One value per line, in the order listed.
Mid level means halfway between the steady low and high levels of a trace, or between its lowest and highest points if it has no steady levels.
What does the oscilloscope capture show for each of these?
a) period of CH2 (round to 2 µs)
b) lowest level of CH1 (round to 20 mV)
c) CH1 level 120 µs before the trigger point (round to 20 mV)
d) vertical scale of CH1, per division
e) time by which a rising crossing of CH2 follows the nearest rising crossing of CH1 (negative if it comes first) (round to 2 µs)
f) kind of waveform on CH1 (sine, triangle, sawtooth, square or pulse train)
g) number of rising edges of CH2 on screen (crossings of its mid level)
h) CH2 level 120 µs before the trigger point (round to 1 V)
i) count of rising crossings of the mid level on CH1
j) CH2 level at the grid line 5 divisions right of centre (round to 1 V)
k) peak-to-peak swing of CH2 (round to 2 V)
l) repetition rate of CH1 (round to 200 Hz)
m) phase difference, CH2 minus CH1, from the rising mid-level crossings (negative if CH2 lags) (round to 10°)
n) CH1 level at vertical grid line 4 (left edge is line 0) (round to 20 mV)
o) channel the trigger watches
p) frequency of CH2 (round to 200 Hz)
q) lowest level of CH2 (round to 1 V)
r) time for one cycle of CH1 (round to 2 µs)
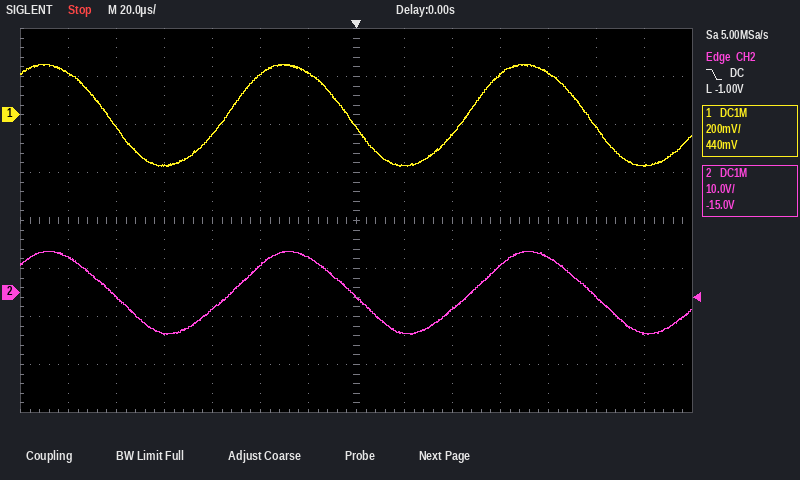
100 µs
-220 mV
180 mV
200 mV
+2 µs
sine
2
7 V
2
-1 V
18 V
10.0 kHz
-10°
-80 mV
CH2
10.0 kHz
-9 V
100 µs
